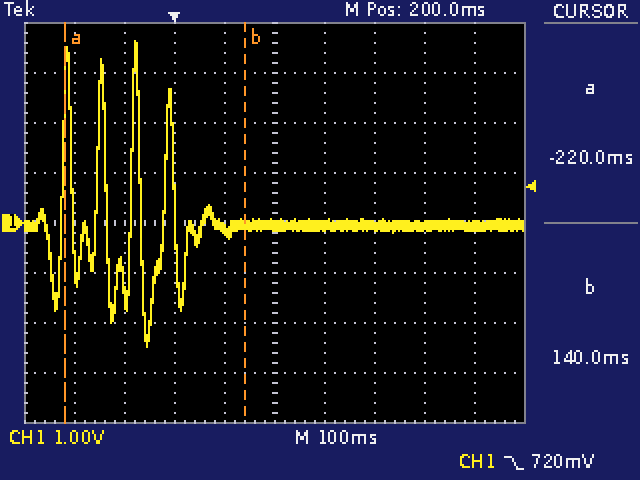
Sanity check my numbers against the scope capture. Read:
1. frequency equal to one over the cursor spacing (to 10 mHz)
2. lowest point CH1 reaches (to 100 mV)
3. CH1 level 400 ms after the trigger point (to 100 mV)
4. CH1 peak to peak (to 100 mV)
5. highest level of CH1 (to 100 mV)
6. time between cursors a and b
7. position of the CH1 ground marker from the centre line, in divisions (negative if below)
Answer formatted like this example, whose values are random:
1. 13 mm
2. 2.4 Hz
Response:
1. 2.78 Hz
2. -2.5 V
3. -100 mV
4. 6.1 V
5. 3.6 V
6. 360 ms
7. 0.0 div
